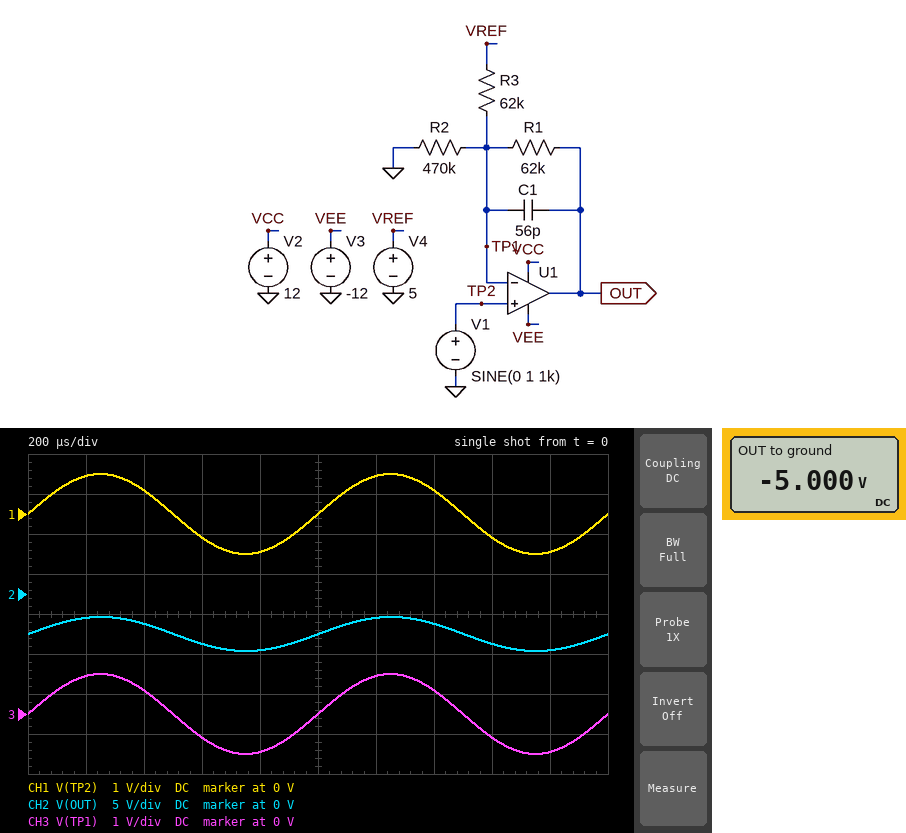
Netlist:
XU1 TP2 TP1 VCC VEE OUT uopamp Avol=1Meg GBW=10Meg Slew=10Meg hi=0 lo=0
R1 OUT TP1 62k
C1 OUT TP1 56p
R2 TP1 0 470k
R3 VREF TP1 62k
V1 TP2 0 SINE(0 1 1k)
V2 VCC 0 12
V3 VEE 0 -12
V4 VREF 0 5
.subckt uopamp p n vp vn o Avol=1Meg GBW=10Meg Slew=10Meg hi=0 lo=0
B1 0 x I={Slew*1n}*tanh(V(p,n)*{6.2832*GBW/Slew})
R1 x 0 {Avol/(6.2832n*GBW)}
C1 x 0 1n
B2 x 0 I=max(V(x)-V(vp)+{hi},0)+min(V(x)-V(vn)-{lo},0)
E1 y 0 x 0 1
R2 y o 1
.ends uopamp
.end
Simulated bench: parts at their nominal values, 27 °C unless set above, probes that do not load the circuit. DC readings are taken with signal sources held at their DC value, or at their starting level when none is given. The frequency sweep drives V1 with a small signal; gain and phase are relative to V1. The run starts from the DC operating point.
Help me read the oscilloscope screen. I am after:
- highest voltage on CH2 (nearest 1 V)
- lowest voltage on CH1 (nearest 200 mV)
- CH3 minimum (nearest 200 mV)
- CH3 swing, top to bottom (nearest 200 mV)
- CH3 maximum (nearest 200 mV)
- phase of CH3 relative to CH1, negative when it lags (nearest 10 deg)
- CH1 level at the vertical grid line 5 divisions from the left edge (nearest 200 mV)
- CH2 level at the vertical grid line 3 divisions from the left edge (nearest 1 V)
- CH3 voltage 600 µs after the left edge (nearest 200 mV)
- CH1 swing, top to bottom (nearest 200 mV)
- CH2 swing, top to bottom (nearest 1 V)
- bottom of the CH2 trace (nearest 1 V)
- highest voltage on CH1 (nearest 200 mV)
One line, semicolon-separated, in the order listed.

-3 V; -1.0 V; -1.0 V; 2.0 V; 1.0 V; 0 deg; 0 V; -6 V; -600 mV; 2.0 V; 4 V; -7 V; 1.0 V
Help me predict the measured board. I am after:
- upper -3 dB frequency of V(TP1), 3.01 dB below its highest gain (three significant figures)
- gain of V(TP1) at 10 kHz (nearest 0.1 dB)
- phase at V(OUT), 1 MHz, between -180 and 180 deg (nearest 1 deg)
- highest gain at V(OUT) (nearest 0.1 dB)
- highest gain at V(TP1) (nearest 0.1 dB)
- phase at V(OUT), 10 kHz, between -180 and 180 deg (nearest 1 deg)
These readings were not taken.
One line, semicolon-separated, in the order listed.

9.95 MHz; 0 dB; -9 deg; 6.6 dB; 0 dB; -7 deg
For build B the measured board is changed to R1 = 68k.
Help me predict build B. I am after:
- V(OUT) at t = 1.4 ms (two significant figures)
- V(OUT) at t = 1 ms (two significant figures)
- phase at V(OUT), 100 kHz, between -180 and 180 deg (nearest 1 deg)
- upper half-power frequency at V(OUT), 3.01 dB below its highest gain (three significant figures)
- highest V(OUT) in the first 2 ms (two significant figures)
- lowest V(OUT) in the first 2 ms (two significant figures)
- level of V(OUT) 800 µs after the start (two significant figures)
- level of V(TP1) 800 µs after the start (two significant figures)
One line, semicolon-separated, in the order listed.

-4.1 V; -5.5 V; -21 deg; 53.4 kHz; -3.2 V; -7.7 V; -7.6 V; -950 mV
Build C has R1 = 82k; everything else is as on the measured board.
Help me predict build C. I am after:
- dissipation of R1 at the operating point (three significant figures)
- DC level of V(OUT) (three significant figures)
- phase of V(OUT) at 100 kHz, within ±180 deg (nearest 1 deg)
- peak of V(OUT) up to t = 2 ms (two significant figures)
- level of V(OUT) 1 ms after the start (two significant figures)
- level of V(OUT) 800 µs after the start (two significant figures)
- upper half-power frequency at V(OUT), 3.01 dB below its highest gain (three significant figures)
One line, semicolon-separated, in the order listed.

533 µW; -6.61 V; -22 deg; -4.1 V; -6.7 V; -9.0 V; 41.7 kHz
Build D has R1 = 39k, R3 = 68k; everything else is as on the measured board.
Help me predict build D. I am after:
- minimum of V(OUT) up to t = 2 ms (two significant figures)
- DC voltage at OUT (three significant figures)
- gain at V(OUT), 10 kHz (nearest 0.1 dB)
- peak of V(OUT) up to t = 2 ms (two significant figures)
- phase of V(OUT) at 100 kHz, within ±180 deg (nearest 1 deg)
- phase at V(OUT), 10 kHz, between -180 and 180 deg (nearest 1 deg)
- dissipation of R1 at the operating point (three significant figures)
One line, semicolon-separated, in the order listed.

-4.5 V; -2.87 V; 4.3 dB; -1.2 V; -15 deg; -3 deg; 211 µW
